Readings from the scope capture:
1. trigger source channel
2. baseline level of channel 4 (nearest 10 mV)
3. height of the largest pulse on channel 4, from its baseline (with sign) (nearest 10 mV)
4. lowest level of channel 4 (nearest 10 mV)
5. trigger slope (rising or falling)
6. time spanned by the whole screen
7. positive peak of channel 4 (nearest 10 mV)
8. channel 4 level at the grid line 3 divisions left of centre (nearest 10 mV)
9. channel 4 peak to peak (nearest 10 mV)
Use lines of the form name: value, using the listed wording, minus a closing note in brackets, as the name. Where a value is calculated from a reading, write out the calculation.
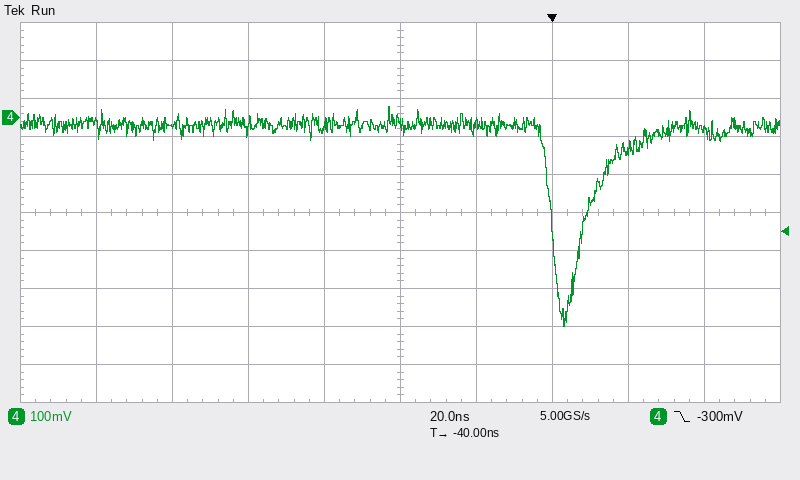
trigger source channel: channel 4
baseline level of channel 4: -20 mV
height of the largest pulse on channel 4, from its baseline (with sign): -550 mV − (-20 mV) = -530 mV
lowest level of channel 4: -550 mV
trigger slope: falling
time spanned by the whole screen: 200 ns
positive peak of channel 4: 30 mV
channel 4 level at the grid line 3 divisions left of centre: -20 mV
channel 4 peak to peak: 30 mV − (-550 mV) = 580 mV
